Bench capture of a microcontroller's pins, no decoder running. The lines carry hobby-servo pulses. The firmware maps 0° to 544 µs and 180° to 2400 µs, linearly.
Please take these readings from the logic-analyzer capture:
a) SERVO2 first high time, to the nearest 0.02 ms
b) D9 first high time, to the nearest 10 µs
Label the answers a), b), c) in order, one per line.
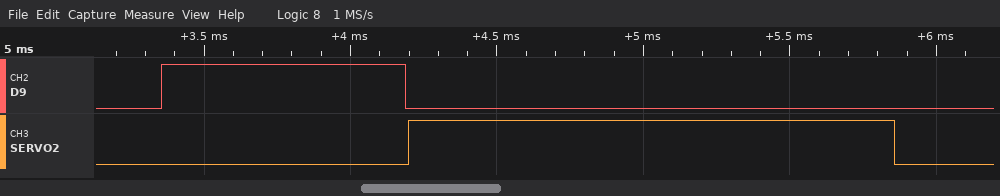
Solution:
a) 1.66 ms
b) 830 µs
